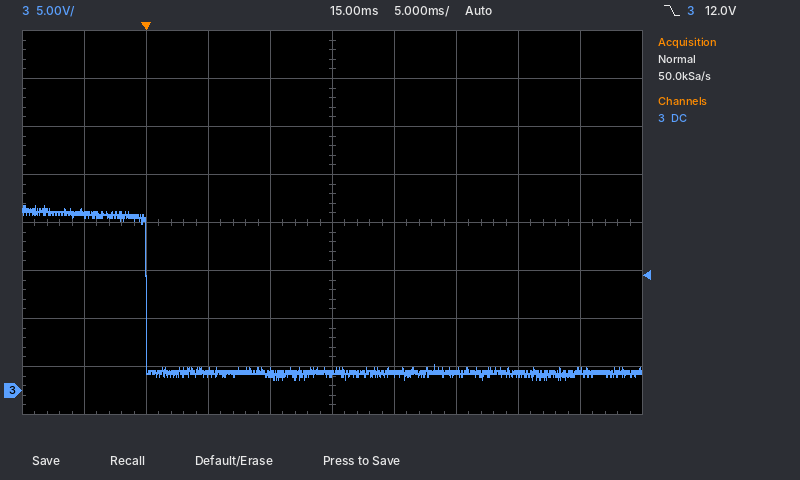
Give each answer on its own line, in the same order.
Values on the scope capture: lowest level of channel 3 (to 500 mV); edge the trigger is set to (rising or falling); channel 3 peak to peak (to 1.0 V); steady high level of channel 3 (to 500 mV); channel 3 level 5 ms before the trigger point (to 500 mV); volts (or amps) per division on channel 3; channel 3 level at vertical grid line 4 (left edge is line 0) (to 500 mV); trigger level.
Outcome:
1.0 V
falling
18.0 V
18.5 V
18.5 V
5 V
2.0 V
12.0 V
